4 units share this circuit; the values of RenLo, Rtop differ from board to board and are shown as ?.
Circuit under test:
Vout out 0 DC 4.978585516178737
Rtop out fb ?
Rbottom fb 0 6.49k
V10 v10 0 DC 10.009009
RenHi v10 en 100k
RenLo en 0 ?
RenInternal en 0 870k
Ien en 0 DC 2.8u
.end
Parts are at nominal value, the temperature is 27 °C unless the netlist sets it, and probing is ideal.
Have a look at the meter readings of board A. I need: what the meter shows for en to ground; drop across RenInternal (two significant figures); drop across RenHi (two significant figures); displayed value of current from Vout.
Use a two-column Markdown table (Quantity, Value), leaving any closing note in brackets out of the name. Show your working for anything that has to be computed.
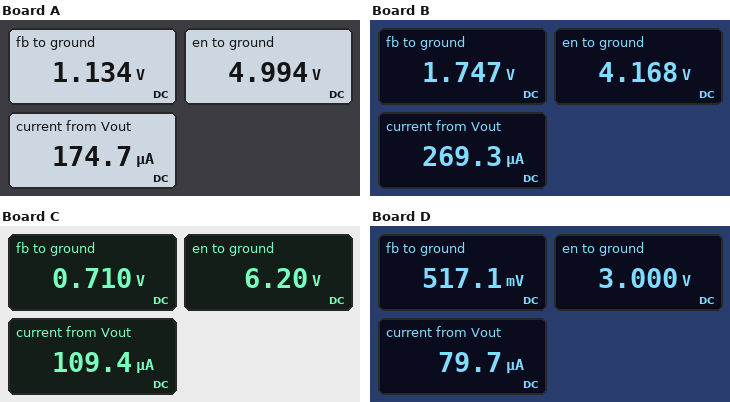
| Quantity | Value |
|---|---|
| what the meter shows for en to ground | 4.994 V |
| drop across RenInternal | 4.994 V = 5.0 V |
| drop across RenHi | 10.01 V - 4.994 V = 5.0 V |
| displayed value of current from Vout | 174.7 µA |
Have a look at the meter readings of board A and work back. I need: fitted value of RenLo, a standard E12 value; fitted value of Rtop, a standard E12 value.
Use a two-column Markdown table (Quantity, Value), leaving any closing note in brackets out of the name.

| Quantity | Value |
|---|---|
| fitted value of RenLo, a standard E12 value | 120 kΩ |
| fitted value of Rtop, a standard E12 value | 22 kΩ |
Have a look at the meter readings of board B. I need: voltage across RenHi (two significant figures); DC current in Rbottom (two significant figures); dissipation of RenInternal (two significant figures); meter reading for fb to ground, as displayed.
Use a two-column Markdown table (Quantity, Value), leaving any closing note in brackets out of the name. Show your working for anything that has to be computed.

| Quantity | Value |
|---|---|
| voltage across RenHi | 10.01 V - 4.168 V = 5.8 V |
| DC current in Rbottom | (1.747 V) / 6.49 kΩ = 270 µA |
| dissipation of RenInternal | (4.168 V)^2 / 870 kΩ = 20 µW |
| meter reading for fb to ground, as displayed | 1.747 V |
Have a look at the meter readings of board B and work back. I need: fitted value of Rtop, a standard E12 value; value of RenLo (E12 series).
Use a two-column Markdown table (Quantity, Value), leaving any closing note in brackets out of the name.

| Quantity | Value |
|---|---|
| fitted value of Rtop, a standard E12 value | 12 kΩ |
| value of RenLo | 82 kΩ |
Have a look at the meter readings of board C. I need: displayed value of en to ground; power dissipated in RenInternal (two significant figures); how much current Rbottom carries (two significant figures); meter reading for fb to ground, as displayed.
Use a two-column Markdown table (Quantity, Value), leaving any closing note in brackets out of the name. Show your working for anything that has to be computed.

| Quantity | Value |
|---|---|
| displayed value of en to ground | 6.20 V |
| power dissipated in RenInternal | (6.2 V)^2 / 870 kΩ = 44 µW |
| how much current Rbottom carries | (710 mV) / 6.49 kΩ = 110 µA |
| meter reading for fb to ground, as displayed | 0.710 V |
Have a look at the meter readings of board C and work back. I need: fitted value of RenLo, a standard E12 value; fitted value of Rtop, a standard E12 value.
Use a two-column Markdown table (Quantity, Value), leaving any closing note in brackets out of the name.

| Quantity | Value |
|---|---|
| fitted value of RenLo, a standard E12 value | 220 kΩ |
| fitted value of Rtop, a standard E12 value | 39 kΩ |
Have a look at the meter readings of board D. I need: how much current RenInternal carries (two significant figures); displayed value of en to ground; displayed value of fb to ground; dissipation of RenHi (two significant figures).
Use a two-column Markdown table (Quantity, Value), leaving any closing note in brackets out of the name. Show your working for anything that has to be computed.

| Quantity | Value |
|---|---|
| how much current RenInternal carries | (3 V) / 870 kΩ = 3.4 µA |
| displayed value of en to ground | 3.000 V |
| displayed value of fb to ground | 517.1 mV |
| dissipation of RenHi | (10.01 V - 3 V)^2 / 100 kΩ = 490 µW |
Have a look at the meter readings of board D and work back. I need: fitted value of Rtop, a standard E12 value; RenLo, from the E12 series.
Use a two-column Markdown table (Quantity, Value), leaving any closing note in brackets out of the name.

| Quantity | Value |
|---|---|
| fitted value of Rtop, a standard E12 value | 56 kΩ |
| RenLo, from the E12 series | 47 kΩ |
